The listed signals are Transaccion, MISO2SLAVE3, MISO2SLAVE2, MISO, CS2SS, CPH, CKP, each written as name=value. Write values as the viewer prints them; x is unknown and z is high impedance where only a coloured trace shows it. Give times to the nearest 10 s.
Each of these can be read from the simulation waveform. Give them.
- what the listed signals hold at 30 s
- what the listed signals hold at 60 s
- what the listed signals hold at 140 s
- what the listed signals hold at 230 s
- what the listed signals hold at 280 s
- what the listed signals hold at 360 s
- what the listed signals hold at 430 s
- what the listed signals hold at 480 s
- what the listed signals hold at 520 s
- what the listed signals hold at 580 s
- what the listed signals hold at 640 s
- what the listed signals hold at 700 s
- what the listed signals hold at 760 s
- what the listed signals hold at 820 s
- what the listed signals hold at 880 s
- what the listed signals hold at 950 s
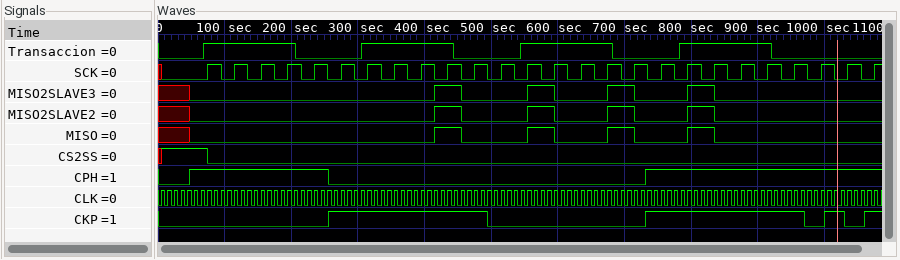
Transaccion=0, MISO2SLAVE3=x, MISO2SLAVE2=x, MISO=x, CS2SS=1, CPH=0, CKP=0
Transaccion=0, MISO2SLAVE3=0, MISO2SLAVE2=0, MISO=0, CS2SS=1, CPH=1, CKP=0
Transaccion=1, MISO2SLAVE3=0, MISO2SLAVE2=0, MISO=0, CS2SS=0, CPH=1, CKP=0
Transaccion=0, MISO2SLAVE3=0, MISO2SLAVE2=0, MISO=0, CS2SS=0, CPH=1, CKP=0
Transaccion=0, MISO2SLAVE3=0, MISO2SLAVE2=0, MISO=0, CS2SS=0, CPH=0, CKP=1
Transaccion=1, MISO2SLAVE3=0, MISO2SLAVE2=0, MISO=0, CS2SS=0, CPH=0, CKP=1
Transaccion=1, MISO2SLAVE3=1, MISO2SLAVE2=1, MISO=1, CS2SS=0, CPH=0, CKP=1
Transaccion=0, MISO2SLAVE3=0, MISO2SLAVE2=0, MISO=0, CS2SS=0, CPH=0, CKP=1
Transaccion=0, MISO2SLAVE3=0, MISO2SLAVE2=0, MISO=0, CS2SS=0, CPH=0, CKP=0
Transaccion=1, MISO2SLAVE3=1, MISO2SLAVE2=1, MISO=1, CS2SS=0, CPH=0, CKP=0
Transaccion=1, MISO2SLAVE3=0, MISO2SLAVE2=0, MISO=0, CS2SS=0, CPH=0, CKP=0
Transaccion=0, MISO2SLAVE3=1, MISO2SLAVE2=1, MISO=1, CS2SS=0, CPH=0, CKP=0
Transaccion=0, MISO2SLAVE3=0, MISO2SLAVE2=0, MISO=0, CS2SS=0, CPH=1, CKP=1
Transaccion=1, MISO2SLAVE3=1, MISO2SLAVE2=1, MISO=1, CS2SS=0, CPH=1, CKP=1
Transaccion=1, MISO2SLAVE3=0, MISO2SLAVE2=0, MISO=0, CS2SS=0, CPH=1, CKP=1
Transaccion=0, MISO2SLAVE3=0, MISO2SLAVE2=0, MISO=0, CS2SS=0, CPH=1, CKP=1
